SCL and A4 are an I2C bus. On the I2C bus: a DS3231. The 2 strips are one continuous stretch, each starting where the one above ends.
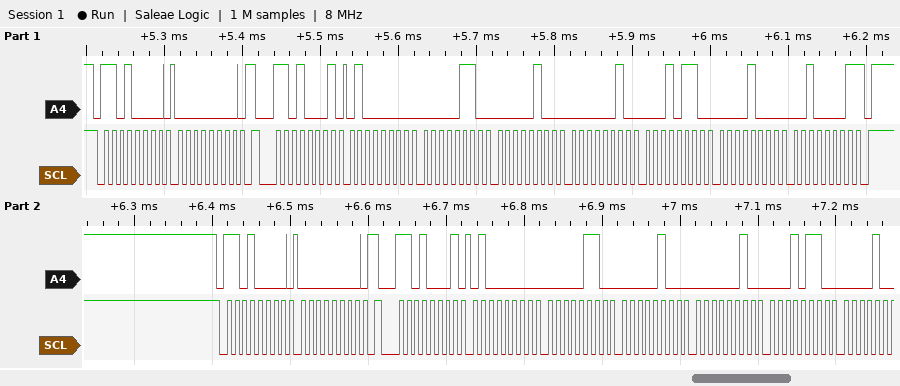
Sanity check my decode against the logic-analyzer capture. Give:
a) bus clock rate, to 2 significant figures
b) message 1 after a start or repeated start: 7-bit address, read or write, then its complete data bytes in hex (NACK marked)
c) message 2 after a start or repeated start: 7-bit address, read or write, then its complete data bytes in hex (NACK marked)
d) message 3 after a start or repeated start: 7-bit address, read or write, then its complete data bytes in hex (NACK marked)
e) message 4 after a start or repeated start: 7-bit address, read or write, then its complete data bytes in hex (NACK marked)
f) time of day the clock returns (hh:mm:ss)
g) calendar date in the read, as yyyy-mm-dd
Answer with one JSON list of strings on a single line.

["100 kHz", "0x68 write: 00", "0x68 read: 40 06 04 02 16 08 21 NACK", "0x68 write: 00", "0x68 read: 40 06 04 02 16", "04:06:40", "2021-08-16"]
